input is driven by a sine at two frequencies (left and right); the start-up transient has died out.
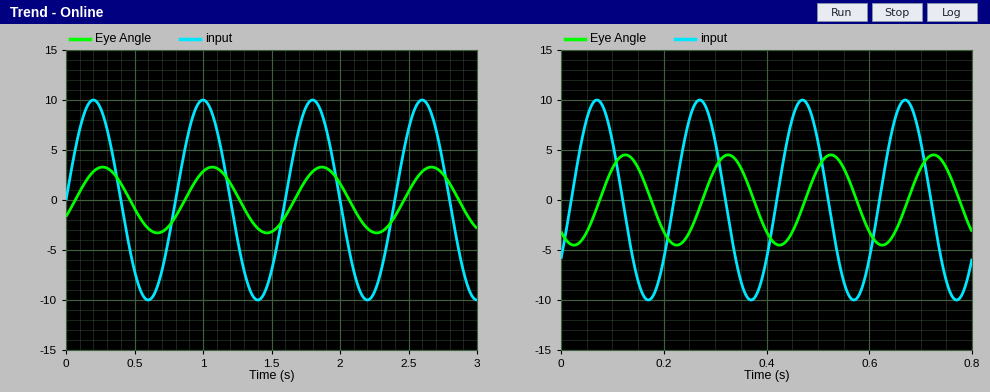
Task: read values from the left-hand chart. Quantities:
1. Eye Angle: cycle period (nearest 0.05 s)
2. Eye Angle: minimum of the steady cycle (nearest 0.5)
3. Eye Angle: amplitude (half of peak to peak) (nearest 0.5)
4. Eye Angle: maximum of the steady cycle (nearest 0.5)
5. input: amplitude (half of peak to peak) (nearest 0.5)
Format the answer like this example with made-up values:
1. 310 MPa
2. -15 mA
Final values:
1. 0.80 s
2. -3.5
3. 3.5
4. 3.5
5. 10.0
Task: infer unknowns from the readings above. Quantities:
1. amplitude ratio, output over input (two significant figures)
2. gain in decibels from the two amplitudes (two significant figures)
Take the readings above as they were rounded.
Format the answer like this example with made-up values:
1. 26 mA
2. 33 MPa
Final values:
1. 0.35
2. -9.1 dB
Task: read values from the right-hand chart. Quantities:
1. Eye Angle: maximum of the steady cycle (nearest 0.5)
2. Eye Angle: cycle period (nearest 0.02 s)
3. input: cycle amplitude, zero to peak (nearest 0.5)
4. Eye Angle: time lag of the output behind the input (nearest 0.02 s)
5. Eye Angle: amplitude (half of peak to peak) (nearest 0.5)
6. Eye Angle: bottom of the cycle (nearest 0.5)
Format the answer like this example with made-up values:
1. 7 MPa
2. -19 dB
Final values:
1. 4.5
2. 0.20 s
3. 10.0
4. 0.06 s
5. 4.5
6. -4.5
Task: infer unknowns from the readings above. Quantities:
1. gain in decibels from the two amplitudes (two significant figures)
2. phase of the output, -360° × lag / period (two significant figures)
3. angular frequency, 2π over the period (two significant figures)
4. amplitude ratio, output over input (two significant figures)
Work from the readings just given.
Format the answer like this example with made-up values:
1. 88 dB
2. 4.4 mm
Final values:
1. -6.9 dB
2. -110°
3. 31 rad/s
4. 0.45
